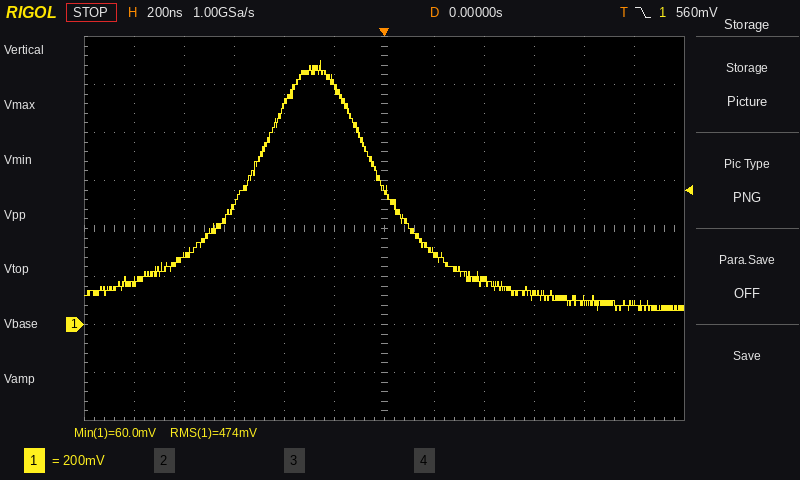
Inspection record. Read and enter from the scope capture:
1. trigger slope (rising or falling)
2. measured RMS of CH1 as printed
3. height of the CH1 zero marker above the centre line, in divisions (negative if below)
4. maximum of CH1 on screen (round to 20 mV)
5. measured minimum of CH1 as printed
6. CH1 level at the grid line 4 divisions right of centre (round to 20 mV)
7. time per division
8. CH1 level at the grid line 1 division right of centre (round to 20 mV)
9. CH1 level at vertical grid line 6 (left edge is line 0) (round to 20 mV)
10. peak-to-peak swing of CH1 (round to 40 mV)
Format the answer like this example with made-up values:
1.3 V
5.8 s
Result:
falling
474 mV
-2.0 div
1.10 V
60.0 mV
100 mV
200 ns
300 mV
560 mV
1.04 V
